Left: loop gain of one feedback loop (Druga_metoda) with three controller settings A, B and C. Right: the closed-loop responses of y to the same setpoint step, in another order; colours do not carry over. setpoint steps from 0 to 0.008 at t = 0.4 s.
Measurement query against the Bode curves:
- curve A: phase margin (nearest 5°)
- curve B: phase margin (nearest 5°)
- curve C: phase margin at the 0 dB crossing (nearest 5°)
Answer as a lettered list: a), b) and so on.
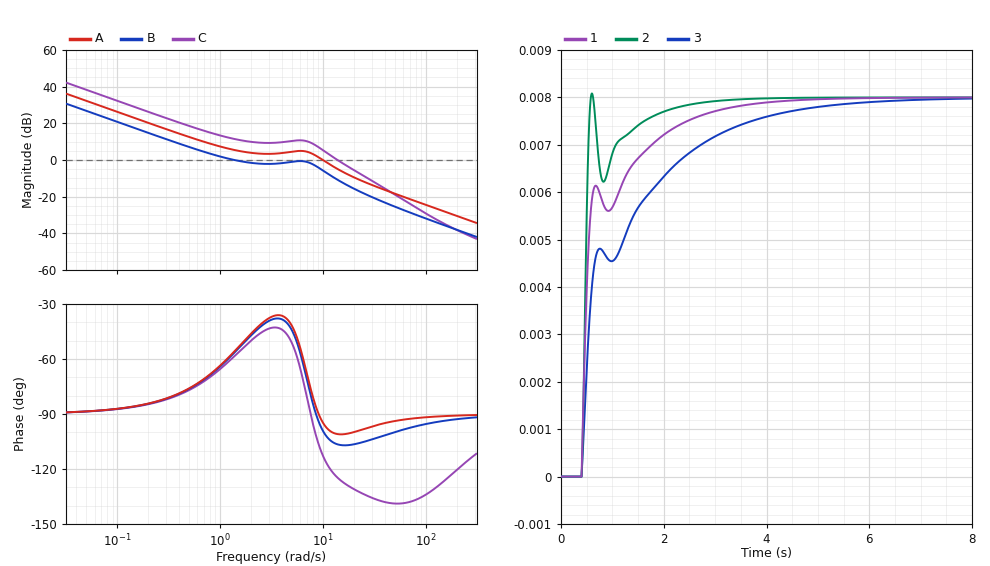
a) 85°
b) 125°
c) 55°
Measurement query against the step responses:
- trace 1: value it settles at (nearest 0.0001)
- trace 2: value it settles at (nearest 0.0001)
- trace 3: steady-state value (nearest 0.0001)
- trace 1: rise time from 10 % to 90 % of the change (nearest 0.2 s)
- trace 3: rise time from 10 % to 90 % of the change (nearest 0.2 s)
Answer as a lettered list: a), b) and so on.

a) 0.0080
b) 0.0080
c) 0.0080
d) 1.6 s
e) 2.6 s
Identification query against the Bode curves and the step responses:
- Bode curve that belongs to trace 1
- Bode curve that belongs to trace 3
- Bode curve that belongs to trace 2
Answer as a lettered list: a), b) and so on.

a) A
b) B
c) C
